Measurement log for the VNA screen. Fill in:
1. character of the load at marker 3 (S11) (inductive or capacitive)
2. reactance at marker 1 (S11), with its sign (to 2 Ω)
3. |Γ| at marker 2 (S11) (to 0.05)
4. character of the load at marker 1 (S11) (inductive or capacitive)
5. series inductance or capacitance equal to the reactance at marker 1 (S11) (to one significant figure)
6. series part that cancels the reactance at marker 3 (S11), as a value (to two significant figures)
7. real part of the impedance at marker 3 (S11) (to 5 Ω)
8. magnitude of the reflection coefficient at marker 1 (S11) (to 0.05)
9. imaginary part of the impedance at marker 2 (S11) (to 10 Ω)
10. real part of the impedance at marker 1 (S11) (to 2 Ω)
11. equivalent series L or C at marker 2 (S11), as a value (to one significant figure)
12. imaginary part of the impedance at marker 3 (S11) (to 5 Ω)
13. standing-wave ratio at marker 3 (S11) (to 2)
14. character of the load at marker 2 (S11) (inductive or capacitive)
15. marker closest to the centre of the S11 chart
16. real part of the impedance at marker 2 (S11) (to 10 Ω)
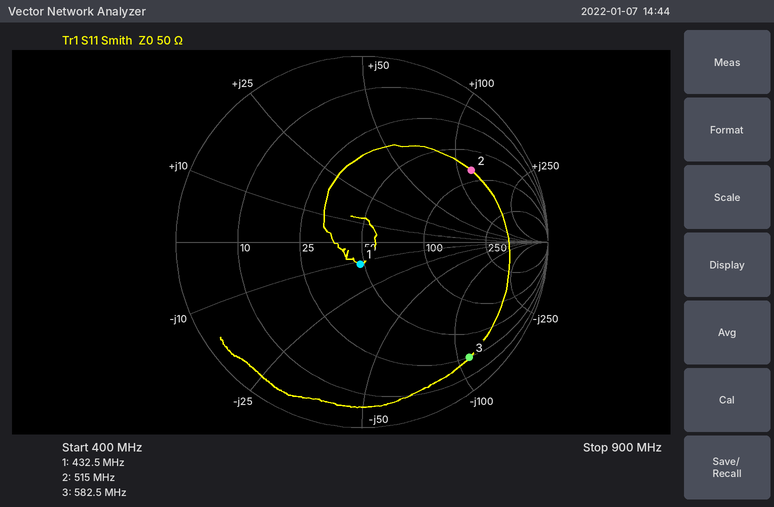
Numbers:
capacitive
-12 Ω
0.70
capacitive
30 pF
30 nH
25 Ω
0.10
+120 Ω
48 Ω
40 nH
-110 Ω
12
inductive
marker 1
80 Ω
